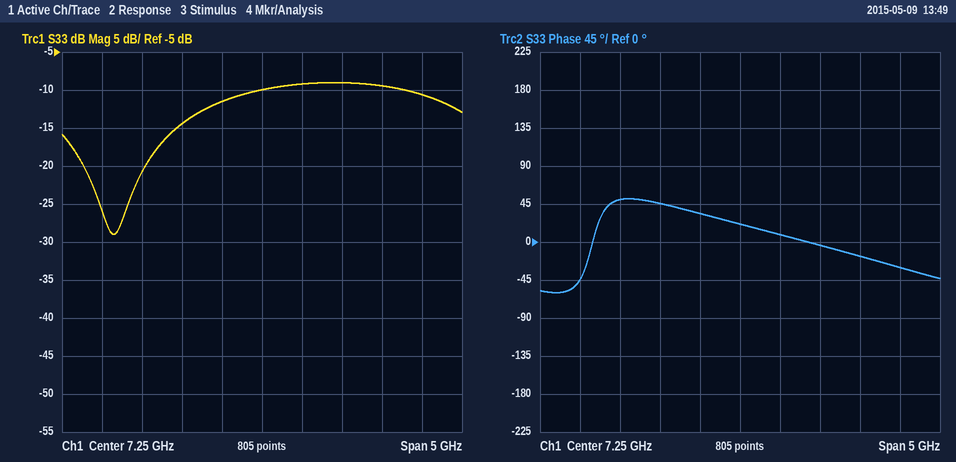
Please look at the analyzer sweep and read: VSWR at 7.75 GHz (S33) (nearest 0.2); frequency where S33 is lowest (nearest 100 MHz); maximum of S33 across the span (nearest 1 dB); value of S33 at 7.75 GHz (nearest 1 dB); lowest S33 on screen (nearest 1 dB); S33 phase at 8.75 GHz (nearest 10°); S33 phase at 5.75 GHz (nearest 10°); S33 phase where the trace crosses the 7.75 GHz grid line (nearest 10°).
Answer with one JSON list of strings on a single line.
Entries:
["2.0", "5.4 GHz", "-9 dB", "-9 dB", "-29 dB", "-20°", "50°", "10°"]
